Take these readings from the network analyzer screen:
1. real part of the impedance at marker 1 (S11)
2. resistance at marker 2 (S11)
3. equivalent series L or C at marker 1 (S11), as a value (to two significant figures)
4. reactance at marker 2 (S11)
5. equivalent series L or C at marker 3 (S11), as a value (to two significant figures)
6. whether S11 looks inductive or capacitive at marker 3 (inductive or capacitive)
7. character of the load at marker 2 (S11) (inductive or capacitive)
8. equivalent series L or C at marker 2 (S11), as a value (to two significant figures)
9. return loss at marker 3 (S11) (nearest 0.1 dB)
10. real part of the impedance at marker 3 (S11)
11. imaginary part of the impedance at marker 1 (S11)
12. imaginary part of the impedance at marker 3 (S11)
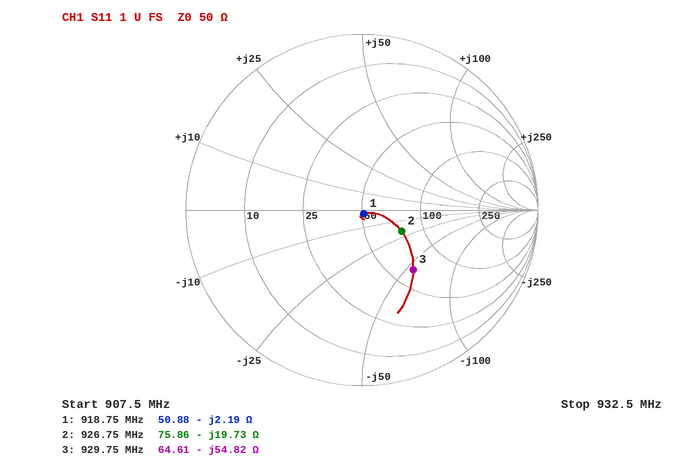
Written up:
50.88 Ω
75.86 Ω
79 pF
-19.73 Ω
3.1 pF
capacitive
capacitive
8.7 pF
7.0 dB
64.61 Ω
-2.19 Ω
-54.82 Ω
